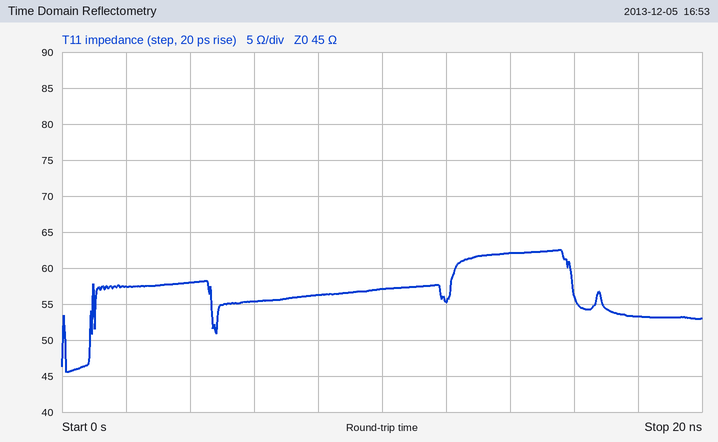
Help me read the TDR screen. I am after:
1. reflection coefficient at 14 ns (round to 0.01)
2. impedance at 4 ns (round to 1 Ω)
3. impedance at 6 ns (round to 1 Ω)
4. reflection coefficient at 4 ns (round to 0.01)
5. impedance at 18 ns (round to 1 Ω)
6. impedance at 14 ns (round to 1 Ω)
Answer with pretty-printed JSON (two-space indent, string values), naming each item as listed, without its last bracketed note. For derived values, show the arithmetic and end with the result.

{
  "reflection coefficient at 14 ns": "(62 − 45)/(62 + 45) ≈ +0.16",
  "impedance at 4 ns": "58 Ω",
  "impedance at 6 ns": "55 Ω",
  "reflection coefficient at 4 ns": "(58 − 45)/(58 + 45) ≈ +0.13",
  "impedance at 18 ns": "53 Ω",
  "impedance at 14 ns": "62 Ω"
}
